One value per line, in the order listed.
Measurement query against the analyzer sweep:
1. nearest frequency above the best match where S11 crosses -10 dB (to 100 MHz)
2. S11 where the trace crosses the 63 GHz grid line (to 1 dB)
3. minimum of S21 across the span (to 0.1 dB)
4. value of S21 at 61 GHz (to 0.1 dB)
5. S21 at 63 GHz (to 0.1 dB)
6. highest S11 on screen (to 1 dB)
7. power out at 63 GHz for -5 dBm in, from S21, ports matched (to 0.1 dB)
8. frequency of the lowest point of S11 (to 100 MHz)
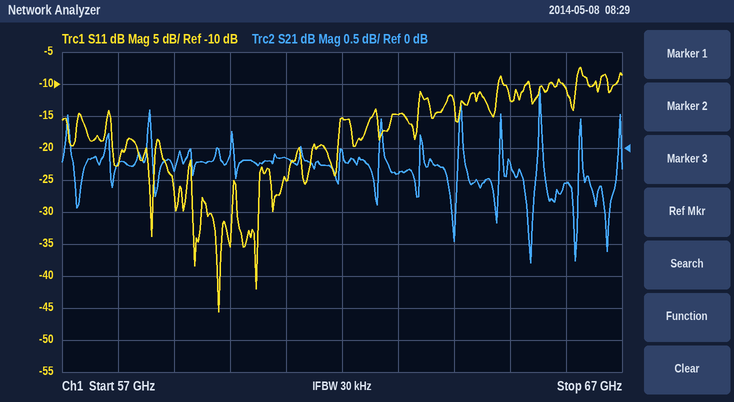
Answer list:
64.8 GHz
-15 dB
-1.8 dB
-0.2 dB
-0.4 dB
-7 dB
-5.4 dBm
59.8 GHz
